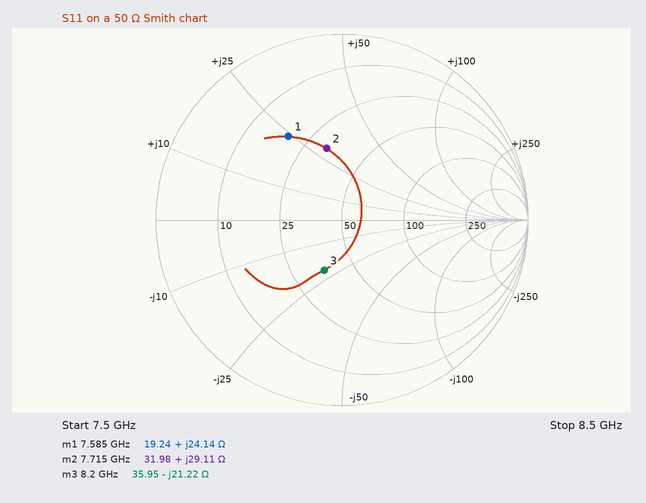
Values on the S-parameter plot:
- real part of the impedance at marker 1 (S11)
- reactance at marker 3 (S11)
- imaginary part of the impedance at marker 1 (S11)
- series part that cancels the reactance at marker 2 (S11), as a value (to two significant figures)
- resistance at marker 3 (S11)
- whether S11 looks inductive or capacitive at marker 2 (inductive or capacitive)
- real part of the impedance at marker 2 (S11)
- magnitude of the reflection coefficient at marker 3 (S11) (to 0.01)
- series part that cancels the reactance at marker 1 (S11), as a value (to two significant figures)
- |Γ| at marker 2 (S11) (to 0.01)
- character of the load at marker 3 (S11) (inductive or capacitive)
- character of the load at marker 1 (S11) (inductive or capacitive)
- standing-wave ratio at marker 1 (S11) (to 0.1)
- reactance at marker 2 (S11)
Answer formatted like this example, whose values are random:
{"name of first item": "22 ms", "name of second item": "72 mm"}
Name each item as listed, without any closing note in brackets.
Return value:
{"real part of the impedance at marker 1": "19.24 Ω", "reactance at marker 3": "-21.22 Ω", "imaginary part of the impedance at marker 1": "+24.14 Ω", "series part that cancels the reactance at marker 2 (S11), as a value": "710 fF", "resistance at marker 3": "35.95 Ω", "whether S11 looks inductive or capacitive at marker 2": "inductive", "real part of the impedance at marker 2": "31.98 Ω", "magnitude of the reflection coefficient at marker 3 (S11)": "0.29", "series part that cancels the reactance at marker 1 (S11), as a value": "870 fF", "|Γ| at marker 2 (S11)": "0.39", "character of the load at marker 3 (S11)": "capacitive", "character of the load at marker 1 (S11)": "inductive", "standing-wave ratio at marker 1 (S11)": "3.3", "reactance at marker 2": "+29.11 Ω"}
